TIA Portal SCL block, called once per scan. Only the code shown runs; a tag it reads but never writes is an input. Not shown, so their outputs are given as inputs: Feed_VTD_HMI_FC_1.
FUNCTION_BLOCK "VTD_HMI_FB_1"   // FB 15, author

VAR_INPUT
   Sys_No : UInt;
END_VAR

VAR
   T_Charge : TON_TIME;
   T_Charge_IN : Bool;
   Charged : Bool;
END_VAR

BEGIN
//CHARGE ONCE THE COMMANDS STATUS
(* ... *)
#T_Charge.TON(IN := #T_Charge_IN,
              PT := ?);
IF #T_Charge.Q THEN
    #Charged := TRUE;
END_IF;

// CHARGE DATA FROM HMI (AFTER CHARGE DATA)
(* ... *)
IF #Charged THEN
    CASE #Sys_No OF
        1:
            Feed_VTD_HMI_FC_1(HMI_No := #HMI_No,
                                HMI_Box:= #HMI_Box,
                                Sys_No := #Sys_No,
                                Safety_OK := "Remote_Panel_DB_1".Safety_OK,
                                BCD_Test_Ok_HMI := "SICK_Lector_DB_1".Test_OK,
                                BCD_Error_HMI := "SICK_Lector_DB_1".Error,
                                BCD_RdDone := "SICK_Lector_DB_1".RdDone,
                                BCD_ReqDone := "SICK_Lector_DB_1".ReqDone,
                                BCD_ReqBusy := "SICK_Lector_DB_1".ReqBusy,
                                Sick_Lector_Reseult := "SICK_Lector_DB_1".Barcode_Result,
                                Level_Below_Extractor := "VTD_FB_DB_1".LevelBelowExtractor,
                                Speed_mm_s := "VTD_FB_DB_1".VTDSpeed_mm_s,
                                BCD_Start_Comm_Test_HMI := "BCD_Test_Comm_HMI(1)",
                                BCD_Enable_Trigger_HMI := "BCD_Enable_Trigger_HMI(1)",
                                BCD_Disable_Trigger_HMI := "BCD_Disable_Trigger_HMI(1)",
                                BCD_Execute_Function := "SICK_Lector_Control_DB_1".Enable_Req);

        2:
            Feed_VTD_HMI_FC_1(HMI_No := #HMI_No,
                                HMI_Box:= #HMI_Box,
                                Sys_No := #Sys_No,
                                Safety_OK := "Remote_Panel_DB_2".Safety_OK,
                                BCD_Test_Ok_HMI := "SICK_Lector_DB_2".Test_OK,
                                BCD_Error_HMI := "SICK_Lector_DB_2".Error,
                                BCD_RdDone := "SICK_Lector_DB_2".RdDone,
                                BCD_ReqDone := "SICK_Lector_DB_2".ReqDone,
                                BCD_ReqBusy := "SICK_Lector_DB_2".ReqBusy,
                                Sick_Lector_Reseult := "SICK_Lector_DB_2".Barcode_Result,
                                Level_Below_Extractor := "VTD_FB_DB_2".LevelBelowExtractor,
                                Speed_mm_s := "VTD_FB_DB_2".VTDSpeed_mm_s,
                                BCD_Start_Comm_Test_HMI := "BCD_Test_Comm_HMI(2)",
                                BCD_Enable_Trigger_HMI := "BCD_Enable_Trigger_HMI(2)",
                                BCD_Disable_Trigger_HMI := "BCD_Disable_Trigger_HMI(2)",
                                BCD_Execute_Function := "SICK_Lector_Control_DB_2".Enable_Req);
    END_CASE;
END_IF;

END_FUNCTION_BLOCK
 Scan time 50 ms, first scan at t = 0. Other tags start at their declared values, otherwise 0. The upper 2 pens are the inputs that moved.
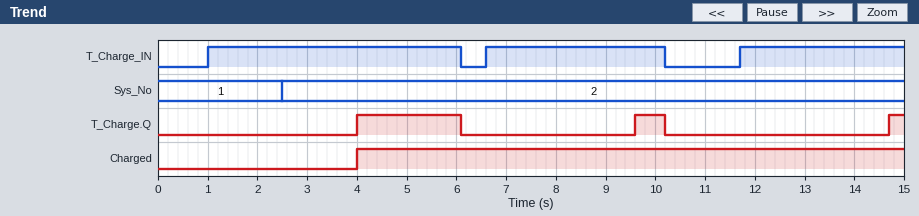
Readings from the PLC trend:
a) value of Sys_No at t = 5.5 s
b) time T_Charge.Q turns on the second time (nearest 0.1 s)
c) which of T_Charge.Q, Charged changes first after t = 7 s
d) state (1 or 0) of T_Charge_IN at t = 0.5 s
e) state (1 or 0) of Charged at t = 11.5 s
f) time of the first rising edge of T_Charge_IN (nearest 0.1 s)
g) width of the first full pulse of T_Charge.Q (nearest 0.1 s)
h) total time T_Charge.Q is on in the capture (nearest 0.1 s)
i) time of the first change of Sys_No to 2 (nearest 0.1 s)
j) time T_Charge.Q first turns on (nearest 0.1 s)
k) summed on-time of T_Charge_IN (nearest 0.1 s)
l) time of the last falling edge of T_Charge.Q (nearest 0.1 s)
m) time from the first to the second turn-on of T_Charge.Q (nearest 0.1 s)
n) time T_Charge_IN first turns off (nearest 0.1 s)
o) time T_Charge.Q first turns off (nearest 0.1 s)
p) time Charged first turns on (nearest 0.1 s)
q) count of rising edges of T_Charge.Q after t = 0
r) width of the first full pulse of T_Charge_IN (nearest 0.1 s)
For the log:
2
9.6 s
T_Charge.Q
0
1
1.0 s
2.1 s
3.0 s
2.5 s
4.0 s
12.0 s
10.2 s
5.6 s
6.1 s
6.1 s
4.0 s
3
5.1 s
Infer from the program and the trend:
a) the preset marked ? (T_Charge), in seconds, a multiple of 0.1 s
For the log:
3.0 s
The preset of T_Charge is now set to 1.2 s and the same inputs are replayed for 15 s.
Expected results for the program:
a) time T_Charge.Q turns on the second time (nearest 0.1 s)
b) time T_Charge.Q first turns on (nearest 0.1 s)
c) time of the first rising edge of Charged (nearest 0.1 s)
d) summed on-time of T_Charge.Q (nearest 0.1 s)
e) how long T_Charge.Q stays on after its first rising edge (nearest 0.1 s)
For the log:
7.8 s
2.2 s
2.2 s
8.4 s
3.9 s
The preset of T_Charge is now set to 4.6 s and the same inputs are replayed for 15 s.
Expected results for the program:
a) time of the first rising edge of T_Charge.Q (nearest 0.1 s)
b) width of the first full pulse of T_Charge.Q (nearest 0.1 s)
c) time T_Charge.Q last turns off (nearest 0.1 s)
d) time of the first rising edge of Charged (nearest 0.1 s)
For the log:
5.6 s
0.5 s
6.1 s
5.6 s
